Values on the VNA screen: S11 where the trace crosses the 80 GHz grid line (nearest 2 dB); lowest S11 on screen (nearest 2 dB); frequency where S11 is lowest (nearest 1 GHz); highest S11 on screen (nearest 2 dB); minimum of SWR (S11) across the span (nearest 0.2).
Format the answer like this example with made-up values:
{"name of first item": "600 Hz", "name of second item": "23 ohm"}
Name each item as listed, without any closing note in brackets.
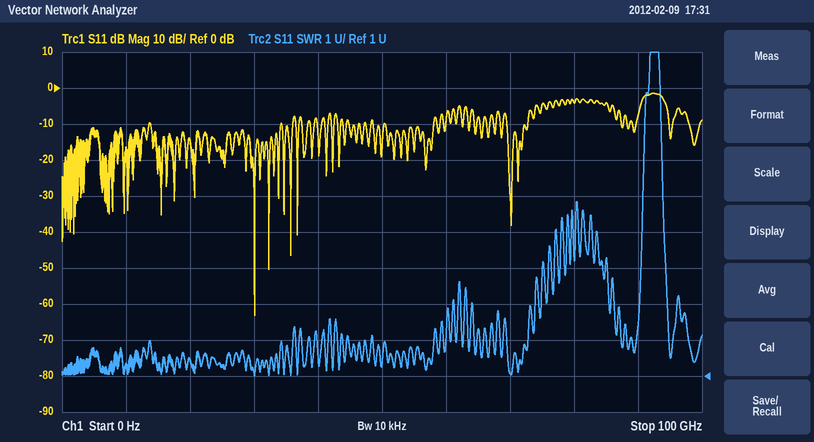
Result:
{"S11 where the trace crosses the 80 GHz grid line": "-4 dB", "lowest S11 on screen": "-64 dB", "frequency where S11 is lowest": "30 GHz", "highest S11 on screen": "-2 dB", "minimum of SWR (S11) across the span": "1.0"}
